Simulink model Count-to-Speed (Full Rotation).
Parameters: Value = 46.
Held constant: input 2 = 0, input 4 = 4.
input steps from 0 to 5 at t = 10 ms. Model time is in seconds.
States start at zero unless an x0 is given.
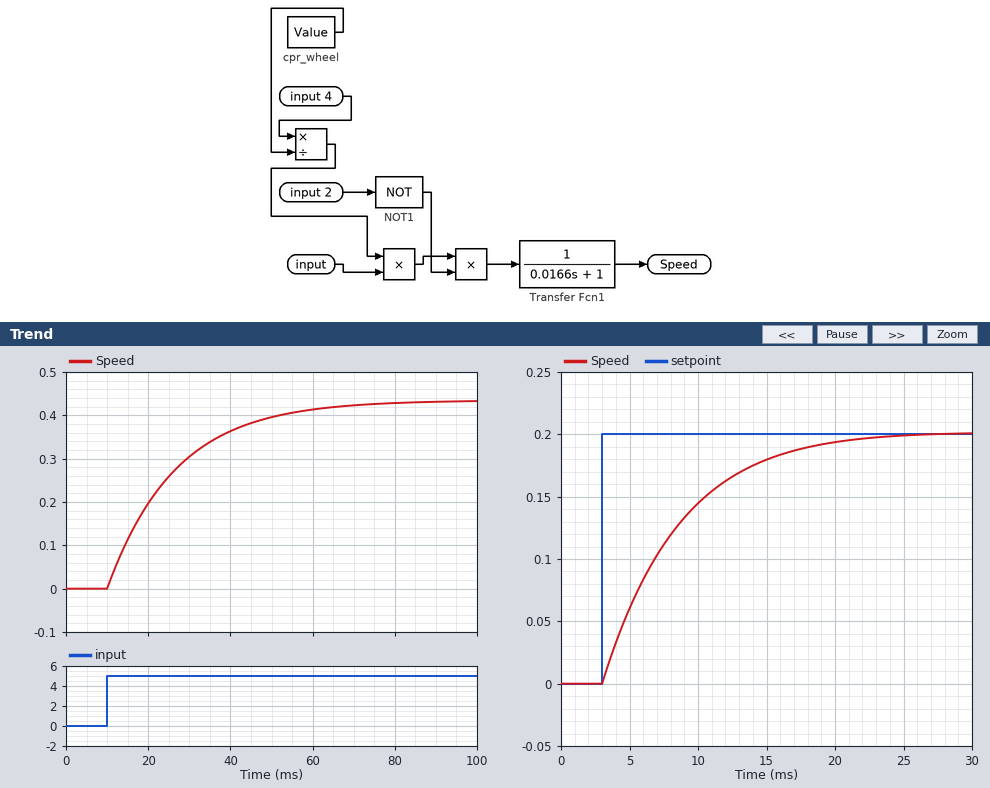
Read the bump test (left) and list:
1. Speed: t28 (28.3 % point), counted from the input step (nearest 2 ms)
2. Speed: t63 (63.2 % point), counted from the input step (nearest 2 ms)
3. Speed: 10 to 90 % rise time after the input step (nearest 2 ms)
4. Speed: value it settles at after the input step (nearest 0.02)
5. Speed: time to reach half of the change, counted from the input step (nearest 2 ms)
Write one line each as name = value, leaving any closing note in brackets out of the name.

Speed: t28 (28.3 % point), counted from the input step = 6 ms
Speed: t63 (63.2 % point), counted from the input step = 16 ms
Speed: 10 to 90 % rise time after the input step = 36 ms
Speed: value it settles at after the input step = 0.44
Speed: time to reach half of the change, counted from the input step = 12 ms
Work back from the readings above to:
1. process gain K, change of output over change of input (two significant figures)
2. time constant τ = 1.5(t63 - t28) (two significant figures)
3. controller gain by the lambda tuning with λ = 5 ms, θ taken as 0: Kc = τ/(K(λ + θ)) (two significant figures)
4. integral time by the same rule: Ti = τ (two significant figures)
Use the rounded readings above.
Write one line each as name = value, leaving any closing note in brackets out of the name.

process gain K, change of output over change of input = 0.088
time constant τ = 1.5(t63 - t28) = 15 ms
controller gain by the lambda tuning with λ = 5 ms, θ taken as 0: Kc = τ/(K(λ + θ)) = 34
integral time by the same rule: Ti = τ = 15 ms
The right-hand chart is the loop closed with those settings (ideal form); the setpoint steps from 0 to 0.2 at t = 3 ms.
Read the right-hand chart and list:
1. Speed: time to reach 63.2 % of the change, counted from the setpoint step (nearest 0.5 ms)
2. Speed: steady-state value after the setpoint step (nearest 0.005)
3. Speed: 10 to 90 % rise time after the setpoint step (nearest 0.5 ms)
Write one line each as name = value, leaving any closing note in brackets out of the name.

Speed: time to reach 63.2 % of the change, counted from the setpoint step = 5.5 ms
Speed: steady-state value after the setpoint step = 0.200
Speed: 10 to 90 % rise time after the setpoint step = 11.5 ms
